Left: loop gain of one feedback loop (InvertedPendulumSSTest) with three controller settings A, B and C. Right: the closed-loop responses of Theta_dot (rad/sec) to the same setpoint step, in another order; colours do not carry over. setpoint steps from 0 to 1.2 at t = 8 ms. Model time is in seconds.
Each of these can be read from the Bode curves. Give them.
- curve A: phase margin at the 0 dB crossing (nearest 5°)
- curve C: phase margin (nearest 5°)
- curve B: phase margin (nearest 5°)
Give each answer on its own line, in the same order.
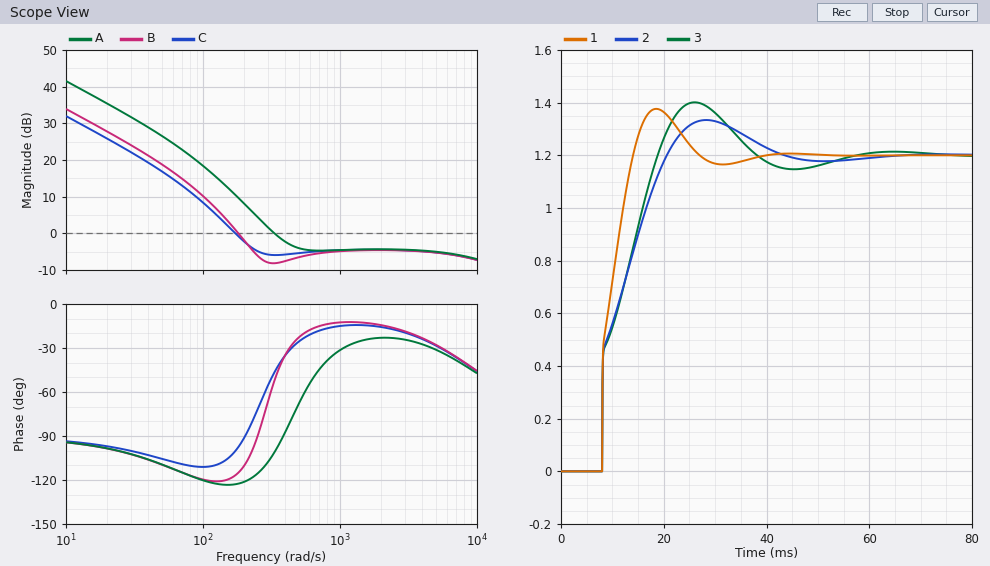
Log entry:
80°
80°
65°
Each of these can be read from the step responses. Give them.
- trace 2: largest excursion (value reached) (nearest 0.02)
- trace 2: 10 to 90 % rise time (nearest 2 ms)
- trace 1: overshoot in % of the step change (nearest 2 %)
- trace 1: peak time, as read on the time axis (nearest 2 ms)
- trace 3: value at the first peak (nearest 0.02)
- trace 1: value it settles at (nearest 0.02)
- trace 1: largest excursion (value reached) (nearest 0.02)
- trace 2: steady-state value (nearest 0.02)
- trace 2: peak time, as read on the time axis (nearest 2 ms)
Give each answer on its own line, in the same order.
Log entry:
1.34
10 ms
14 %
18 ms
1.40
1.20
1.38
1.20
28 ms
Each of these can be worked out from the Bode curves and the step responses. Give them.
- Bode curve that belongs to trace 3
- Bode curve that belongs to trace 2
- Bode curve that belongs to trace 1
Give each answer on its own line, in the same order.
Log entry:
B
C
A
